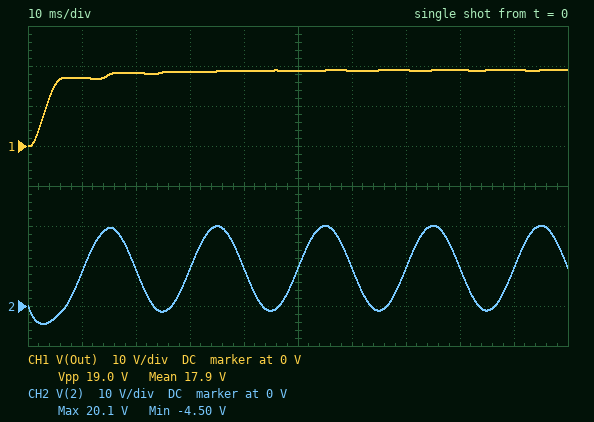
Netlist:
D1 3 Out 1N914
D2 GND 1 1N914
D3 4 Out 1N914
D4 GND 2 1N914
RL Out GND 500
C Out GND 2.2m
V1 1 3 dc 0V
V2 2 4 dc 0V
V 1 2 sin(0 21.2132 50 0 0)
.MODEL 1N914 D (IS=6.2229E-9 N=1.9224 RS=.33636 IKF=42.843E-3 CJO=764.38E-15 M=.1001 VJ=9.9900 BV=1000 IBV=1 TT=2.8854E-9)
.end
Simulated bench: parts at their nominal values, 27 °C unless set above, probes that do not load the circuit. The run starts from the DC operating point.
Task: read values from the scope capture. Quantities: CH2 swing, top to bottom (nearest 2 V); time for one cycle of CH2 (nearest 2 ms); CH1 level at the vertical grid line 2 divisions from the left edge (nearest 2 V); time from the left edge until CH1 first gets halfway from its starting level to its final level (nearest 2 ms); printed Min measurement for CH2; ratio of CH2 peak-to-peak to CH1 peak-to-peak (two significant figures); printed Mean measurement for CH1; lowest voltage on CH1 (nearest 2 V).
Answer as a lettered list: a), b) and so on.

a) 24 V
b) 20 ms
c) 18 V
d) 4 ms
e) -4.50 V
f) 1.3
g) 17.9 V
h) 0 V
